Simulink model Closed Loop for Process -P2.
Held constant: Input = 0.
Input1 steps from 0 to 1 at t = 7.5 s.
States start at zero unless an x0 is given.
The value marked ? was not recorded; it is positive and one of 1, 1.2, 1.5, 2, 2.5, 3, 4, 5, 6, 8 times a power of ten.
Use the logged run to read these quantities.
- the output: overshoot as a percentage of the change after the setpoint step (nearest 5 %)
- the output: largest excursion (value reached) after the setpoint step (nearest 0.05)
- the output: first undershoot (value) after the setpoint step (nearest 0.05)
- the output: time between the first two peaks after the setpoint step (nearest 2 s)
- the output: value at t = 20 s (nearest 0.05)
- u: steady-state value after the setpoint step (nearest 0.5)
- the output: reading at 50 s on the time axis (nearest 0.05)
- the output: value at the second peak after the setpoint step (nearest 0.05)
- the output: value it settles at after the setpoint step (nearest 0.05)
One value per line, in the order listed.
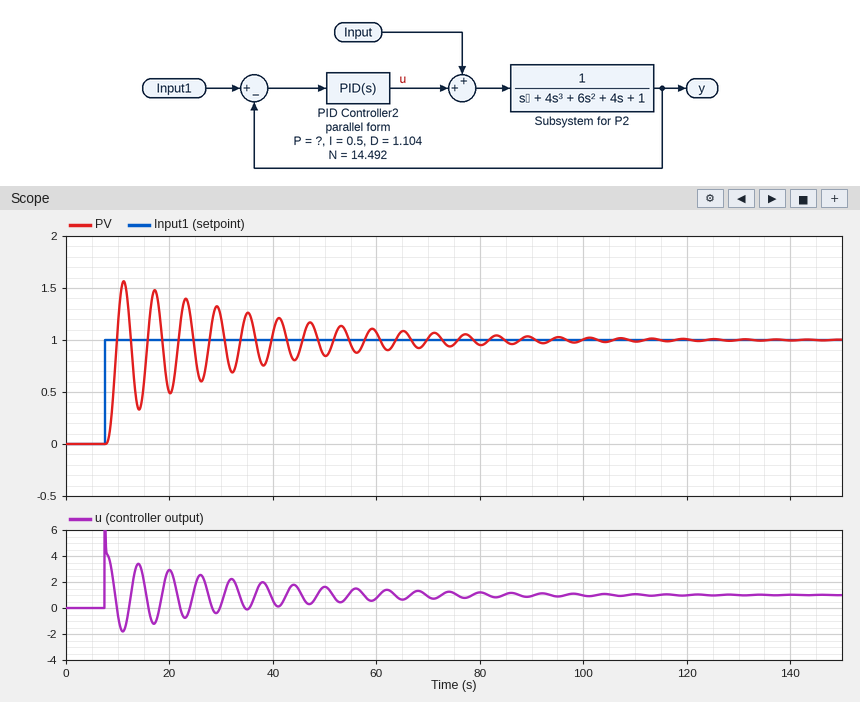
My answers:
55 %
1.55
0.35
6 s
0.50
1.0
0.85
1.50
1.00
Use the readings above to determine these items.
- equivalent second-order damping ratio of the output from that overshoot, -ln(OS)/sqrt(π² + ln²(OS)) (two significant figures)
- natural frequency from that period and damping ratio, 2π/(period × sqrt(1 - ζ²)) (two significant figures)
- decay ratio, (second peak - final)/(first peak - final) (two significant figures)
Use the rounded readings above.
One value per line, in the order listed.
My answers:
0.19
1.1 rad/s
0.91
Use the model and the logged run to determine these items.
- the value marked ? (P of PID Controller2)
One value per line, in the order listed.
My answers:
4
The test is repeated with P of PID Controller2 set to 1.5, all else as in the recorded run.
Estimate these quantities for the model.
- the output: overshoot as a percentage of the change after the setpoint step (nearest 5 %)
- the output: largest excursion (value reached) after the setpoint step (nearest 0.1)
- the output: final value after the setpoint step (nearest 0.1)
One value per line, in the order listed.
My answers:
10 %
1.1
1.0
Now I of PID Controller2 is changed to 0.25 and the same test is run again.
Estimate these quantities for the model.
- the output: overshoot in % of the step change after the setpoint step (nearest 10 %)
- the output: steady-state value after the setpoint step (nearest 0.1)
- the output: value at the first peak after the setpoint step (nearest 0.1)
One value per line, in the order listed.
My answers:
50 %
1.0
1.5
